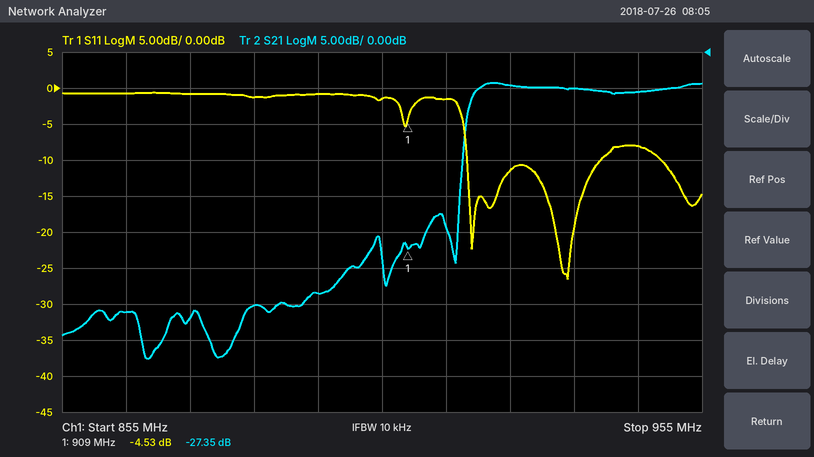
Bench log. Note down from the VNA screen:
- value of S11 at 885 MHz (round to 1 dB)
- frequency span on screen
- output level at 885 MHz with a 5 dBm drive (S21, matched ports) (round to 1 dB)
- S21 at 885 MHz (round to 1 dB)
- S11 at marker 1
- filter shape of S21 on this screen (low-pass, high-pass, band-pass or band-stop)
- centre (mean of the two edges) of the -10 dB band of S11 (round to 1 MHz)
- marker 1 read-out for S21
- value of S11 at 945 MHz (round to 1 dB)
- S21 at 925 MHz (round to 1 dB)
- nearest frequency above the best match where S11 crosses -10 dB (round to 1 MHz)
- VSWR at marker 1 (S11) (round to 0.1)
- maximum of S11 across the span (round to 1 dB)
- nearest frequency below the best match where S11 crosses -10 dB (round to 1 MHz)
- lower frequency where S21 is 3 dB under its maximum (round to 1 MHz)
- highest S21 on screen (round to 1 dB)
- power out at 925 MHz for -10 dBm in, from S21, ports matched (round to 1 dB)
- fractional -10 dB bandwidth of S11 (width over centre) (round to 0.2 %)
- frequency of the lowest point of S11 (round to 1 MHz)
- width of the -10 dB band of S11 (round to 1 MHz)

-1 dB
100 MHz
-30 dBm
-35 dB
-4.53 dB
high-pass
929 MHz
-27.35 dB
-8 dB
-5 dB
939 MHz
3.9
-1 dB
918 MHz
919 MHz
-4 dB
-15 dBm
2.2 %
934 MHz
21 MHz
